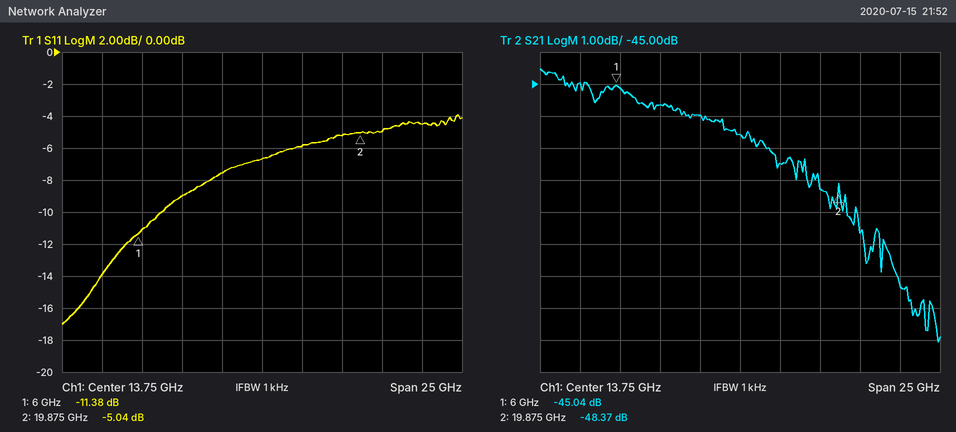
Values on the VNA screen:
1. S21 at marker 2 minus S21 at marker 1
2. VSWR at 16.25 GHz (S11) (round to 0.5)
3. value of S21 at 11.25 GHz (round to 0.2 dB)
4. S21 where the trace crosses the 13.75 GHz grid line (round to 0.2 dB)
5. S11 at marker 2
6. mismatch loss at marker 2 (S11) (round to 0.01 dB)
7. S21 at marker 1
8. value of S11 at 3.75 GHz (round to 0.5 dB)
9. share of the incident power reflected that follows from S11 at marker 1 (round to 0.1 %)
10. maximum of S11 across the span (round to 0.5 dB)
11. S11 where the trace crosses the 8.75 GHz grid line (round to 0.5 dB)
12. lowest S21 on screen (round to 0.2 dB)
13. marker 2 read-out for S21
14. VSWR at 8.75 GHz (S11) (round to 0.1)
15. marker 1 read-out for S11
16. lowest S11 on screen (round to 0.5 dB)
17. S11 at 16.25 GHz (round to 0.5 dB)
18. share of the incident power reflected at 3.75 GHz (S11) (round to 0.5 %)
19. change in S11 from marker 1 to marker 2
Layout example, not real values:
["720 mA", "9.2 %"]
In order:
["-3.33 dB", "3.0", "-46.0 dB", "-46.6 dB", "-5.04 dB", "1.63 dB", "-45.04 dB", "-14.0 dB", "7.3 %", "-4.0 dB", "-9.0 dB", "-53.0 dB", "-48.37 dB", "2.1", "-11.38 dB", "-17.0 dB", "-6.0 dB", "4.0 %", "6.34 dB"]
